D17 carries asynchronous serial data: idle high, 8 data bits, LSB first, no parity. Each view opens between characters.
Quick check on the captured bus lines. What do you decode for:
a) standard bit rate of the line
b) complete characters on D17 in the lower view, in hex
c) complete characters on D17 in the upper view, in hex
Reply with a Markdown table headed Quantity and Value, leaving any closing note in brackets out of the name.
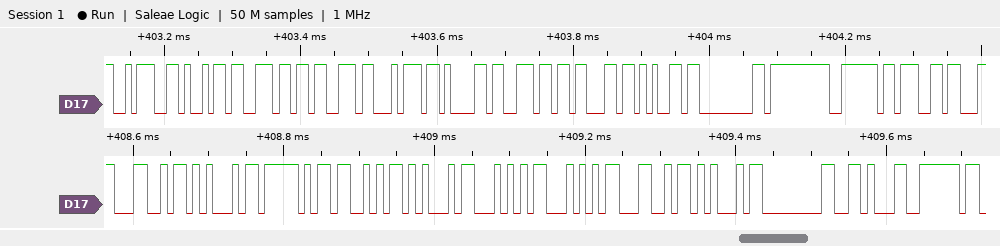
| Quantity | Value |
|---|---|
| standard bit rate of the line | 115200 baud |
| complete characters on D17 in the lower view, in hex | 4C, 45, 5F, 53, 45, 54, 54, 4C, 45, 00, 16, 7E |
| complete characters on D17 in the upper view, in hex | 3A, 69, 6E, 73, 74, 61, 6E, 63, 65, 00, FF, 7E, 67 |
